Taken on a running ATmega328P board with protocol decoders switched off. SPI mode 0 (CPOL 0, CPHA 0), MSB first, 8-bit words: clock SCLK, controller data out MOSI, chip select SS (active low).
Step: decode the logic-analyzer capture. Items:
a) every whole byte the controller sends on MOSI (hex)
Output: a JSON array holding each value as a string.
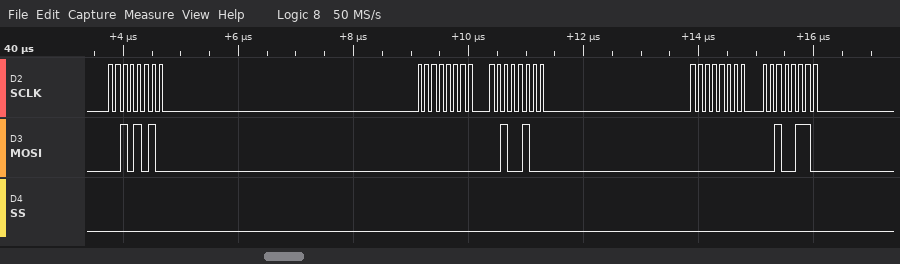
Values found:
["2A 00 24 00 26"]
